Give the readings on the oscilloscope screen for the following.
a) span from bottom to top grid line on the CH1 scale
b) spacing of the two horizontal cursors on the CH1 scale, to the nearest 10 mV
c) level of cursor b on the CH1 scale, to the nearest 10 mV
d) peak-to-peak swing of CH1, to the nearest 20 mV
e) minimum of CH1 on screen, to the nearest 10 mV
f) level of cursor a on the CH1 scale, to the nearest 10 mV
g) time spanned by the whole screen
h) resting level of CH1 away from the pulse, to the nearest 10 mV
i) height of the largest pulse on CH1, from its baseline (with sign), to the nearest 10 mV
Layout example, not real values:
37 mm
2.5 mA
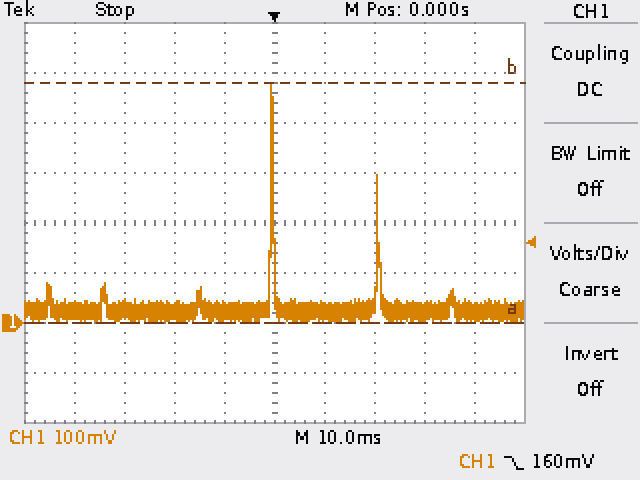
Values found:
800 mV
480 mV
480 mV
480 mV
0 mV
0 mV
100 ms
20 mV
+450 mV
